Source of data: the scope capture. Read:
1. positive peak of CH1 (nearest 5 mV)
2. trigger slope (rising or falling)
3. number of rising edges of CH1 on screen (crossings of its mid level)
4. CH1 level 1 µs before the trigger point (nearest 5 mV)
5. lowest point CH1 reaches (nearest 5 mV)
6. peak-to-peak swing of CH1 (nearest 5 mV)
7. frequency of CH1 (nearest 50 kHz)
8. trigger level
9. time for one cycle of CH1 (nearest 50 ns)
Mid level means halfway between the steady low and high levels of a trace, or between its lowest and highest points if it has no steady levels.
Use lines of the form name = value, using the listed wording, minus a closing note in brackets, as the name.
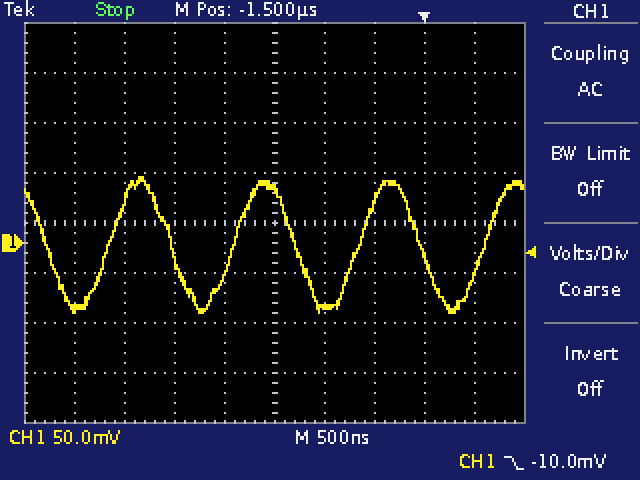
positive peak of CH1 = 65 mV
trigger slope = falling
number of rising edges of CH1 on screen = 4
CH1 level 1 µs before the trigger point = -65 mV
lowest point CH1 reaches = -70 mV
peak-to-peak swing of CH1 = 135 mV
frequency of CH1 = 800 kHz
trigger level = -10.0 mV
time for one cycle of CH1 = 1.25 µs
